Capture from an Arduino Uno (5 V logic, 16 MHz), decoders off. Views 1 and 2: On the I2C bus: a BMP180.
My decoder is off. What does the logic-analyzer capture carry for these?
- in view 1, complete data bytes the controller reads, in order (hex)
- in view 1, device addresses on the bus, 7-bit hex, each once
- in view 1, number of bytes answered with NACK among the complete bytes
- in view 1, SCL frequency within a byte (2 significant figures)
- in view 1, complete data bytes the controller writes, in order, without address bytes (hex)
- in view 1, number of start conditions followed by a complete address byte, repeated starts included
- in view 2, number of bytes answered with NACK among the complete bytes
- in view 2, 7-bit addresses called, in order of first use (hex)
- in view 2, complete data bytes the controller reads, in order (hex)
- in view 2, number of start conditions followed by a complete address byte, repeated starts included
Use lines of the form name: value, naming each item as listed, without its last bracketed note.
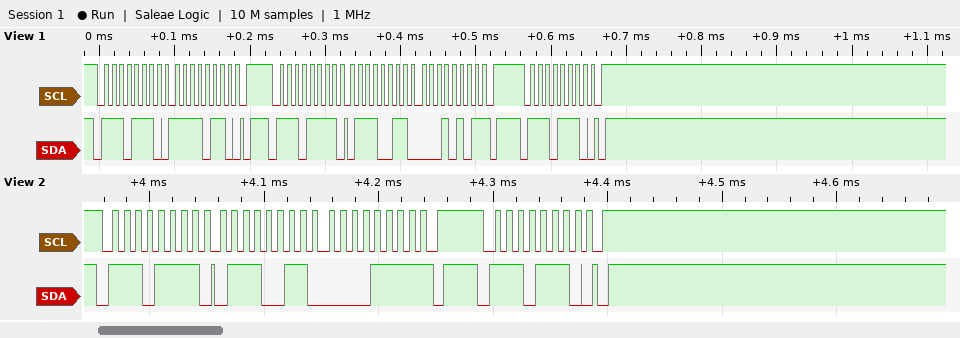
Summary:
in view 1, complete data bytes the controller reads, in order: 73 15
in view 1, device addresses on the bus, 7-bit hex, each once: 0x77
in view 1, number of bytes answered with NACK among the complete bytes: 1
in view 1, SCL frequency within a byte: 100 kHz
in view 1, complete data bytes the controller writes, in order, without address bytes: F6
in view 1, number of start conditions followed by a complete address byte, repeated starts included: 3
in view 2, number of bytes answered with NACK among the complete bytes: 1
in view 2, 7-bit addresses called, in order of first use: 0x77
in view 2, complete data bytes the controller reads, in order: 73 0F
in view 2, number of start conditions followed by a complete address byte, repeated starts included: 2
